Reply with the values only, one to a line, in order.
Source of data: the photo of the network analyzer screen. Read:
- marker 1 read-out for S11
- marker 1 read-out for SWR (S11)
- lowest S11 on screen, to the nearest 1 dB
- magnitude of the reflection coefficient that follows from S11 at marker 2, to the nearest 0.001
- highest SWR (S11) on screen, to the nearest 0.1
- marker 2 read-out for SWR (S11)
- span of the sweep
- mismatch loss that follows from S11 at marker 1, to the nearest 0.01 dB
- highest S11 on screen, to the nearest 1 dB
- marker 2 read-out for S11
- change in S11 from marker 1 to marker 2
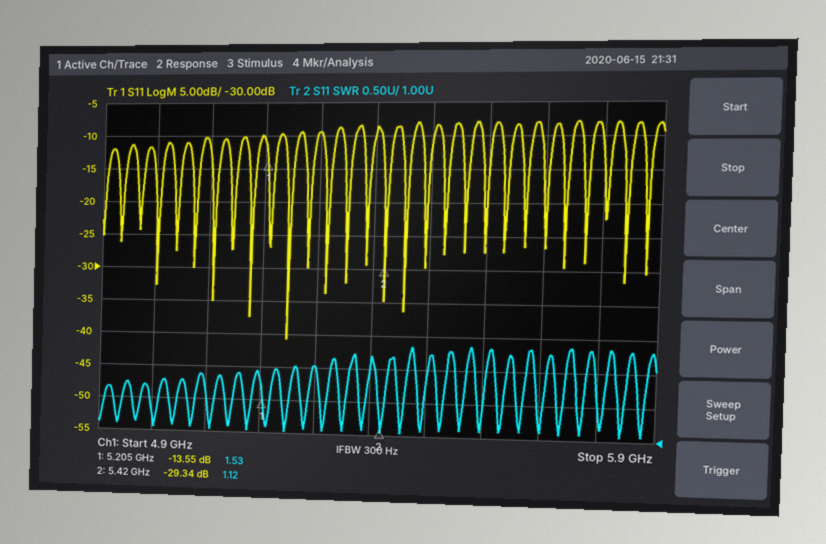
-13.55 dB
1.53
-41 dB
0.034
2.4
1.12
1 GHz
0.20 dB
-8 dB
-29.34 dB
-15.79 dB
